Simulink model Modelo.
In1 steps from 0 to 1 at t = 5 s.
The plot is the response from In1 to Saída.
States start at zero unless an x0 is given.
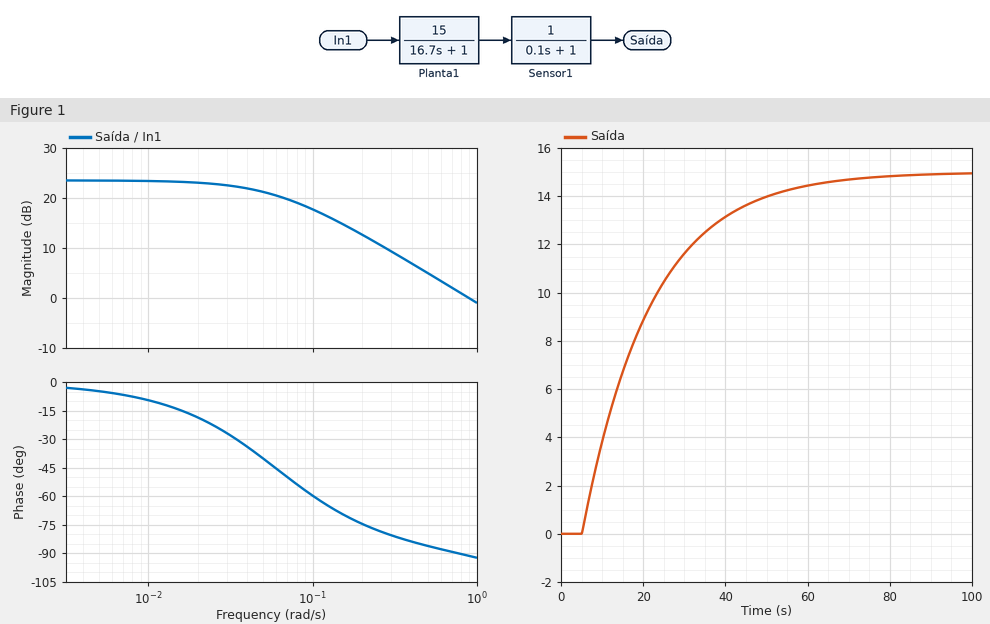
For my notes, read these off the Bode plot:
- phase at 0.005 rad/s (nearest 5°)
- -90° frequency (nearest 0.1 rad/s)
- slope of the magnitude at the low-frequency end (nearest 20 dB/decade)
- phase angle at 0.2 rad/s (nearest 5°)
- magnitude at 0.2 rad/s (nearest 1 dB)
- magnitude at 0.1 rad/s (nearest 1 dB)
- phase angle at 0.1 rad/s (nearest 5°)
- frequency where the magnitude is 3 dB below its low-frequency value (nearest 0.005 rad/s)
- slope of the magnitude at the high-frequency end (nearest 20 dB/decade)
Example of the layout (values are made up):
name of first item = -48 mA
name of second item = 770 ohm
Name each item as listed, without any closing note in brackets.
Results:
phase at 0.005 rad/s = -5°
-90° frequency = 0.8 rad/s
slope of the magnitude at the low-frequency end = 0 dB/decade
phase angle at 0.2 rad/s = -75°
magnitude at 0.2 rad/s = 13 dB
magnitude at 0.1 rad/s = 18 dB
phase angle at 0.1 rad/s = -60°
frequency where the magnitude is 3 dB below its low-frequency value = 0.060 rad/s
slope of the magnitude at the high-frequency end = -20 dB/decade
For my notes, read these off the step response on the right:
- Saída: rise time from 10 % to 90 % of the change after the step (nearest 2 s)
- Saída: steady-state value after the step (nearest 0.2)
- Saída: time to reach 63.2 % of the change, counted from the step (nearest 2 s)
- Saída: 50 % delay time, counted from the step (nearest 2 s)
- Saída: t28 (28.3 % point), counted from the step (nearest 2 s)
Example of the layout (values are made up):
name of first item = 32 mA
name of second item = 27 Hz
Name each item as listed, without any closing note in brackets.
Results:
Saída: rise time from 10 % to 90 % of the change after the step = 36 s
Saída: steady-state value after the step = 15.0
Saída: time to reach 63.2 % of the change, counted from the step = 16 s
Saída: 50 % delay time, counted from the step = 12 s
Saída: t28 (28.3 % point), counted from the step = 6 s
